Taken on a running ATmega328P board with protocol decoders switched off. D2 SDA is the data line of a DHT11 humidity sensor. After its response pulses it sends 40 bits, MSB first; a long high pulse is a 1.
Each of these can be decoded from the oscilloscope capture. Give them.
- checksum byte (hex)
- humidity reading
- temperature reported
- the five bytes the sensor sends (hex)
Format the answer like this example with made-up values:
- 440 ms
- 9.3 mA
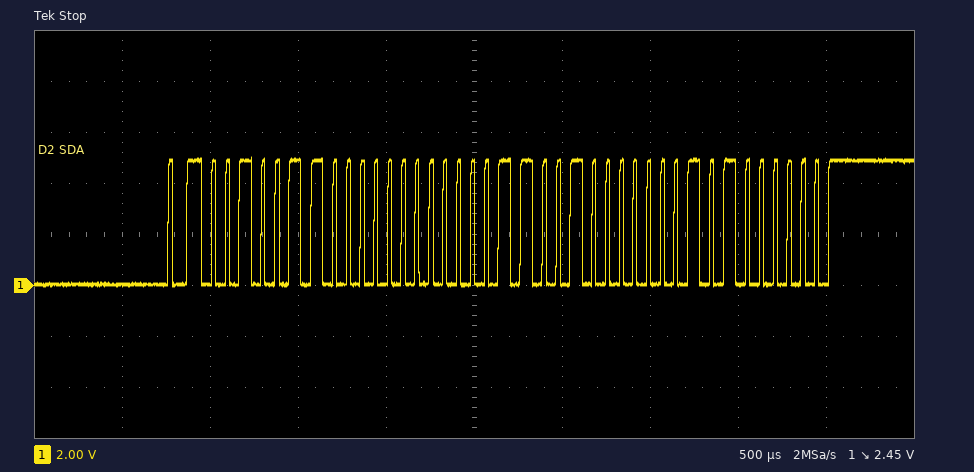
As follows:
- 0x40
- 38 %
- 25.1 °C
- 26 00 19 01 40
